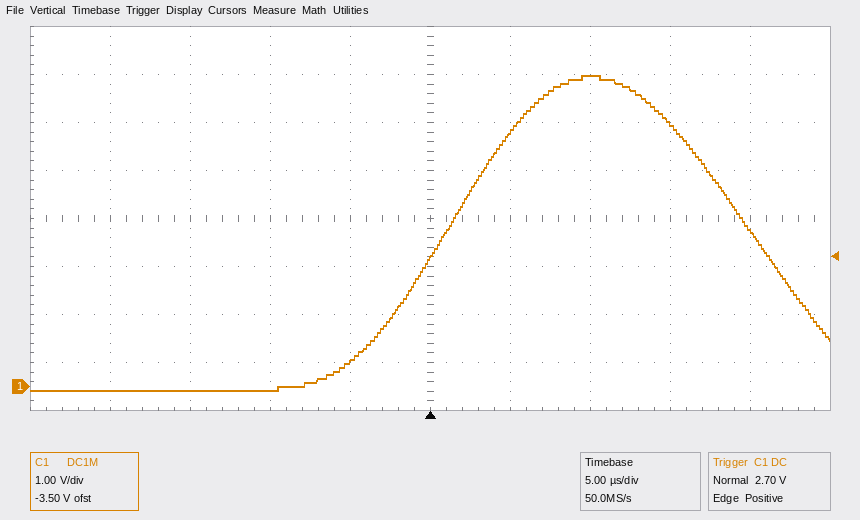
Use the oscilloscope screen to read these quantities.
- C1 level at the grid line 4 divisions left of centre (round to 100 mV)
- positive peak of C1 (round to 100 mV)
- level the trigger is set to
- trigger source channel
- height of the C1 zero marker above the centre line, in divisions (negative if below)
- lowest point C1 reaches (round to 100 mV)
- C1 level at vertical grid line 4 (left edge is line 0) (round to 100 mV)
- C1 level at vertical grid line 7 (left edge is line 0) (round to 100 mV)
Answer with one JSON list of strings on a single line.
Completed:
["-100 mV", "6.5 V", "2.70 V", "C1", "-3.5 div", "-100 mV", "500 mV", "6.5 V"]
